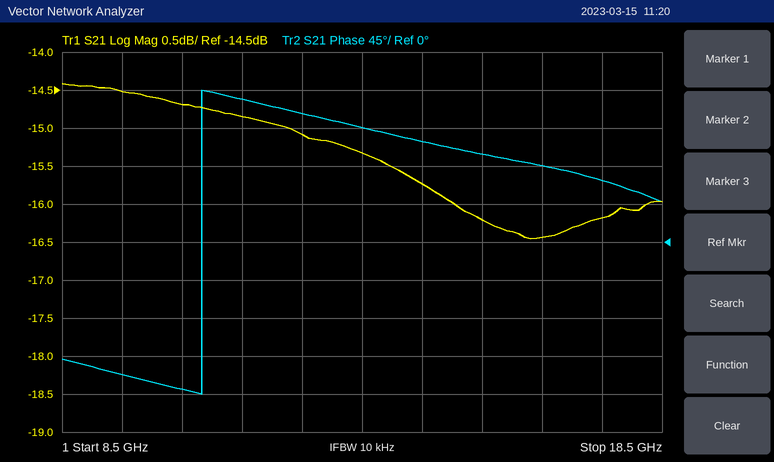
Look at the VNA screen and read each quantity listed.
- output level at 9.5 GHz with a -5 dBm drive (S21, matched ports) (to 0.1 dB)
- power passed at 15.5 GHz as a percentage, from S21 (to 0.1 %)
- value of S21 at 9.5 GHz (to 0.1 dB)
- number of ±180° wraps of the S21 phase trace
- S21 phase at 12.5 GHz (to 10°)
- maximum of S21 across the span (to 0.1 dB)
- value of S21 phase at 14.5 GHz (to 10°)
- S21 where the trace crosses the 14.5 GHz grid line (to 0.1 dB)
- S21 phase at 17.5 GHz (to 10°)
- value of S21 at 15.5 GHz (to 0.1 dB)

-19.5 dBm
2.4 %
-14.5 dB
1
150°
-14.4 dB
120°
-15.7 dB
70°
-16.2 dB
